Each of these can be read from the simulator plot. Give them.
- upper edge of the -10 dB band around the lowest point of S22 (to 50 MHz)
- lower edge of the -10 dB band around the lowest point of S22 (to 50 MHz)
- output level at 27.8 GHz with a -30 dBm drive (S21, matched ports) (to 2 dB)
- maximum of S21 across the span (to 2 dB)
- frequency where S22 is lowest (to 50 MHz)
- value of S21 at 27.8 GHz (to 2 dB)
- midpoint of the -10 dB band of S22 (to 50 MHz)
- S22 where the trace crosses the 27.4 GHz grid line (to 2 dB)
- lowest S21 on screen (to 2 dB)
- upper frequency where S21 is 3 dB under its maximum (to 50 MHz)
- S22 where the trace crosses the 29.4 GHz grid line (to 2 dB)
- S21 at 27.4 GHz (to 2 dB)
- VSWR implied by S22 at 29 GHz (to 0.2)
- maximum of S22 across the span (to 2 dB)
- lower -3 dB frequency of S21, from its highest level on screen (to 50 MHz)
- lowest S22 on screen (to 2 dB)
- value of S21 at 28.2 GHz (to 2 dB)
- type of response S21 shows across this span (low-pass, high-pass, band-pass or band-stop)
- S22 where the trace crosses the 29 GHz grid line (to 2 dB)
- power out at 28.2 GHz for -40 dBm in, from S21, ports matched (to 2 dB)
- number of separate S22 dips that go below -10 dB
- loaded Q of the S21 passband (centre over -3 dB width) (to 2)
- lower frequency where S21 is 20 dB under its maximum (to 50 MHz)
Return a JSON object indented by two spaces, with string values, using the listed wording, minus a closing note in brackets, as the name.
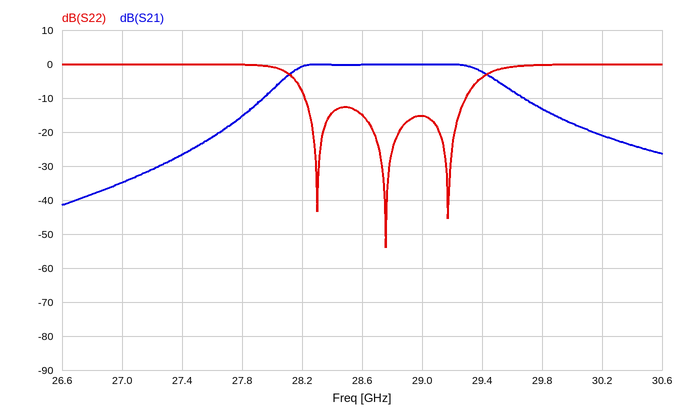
{
  "upper edge of the -10 dB band around the lowest point of S22": "29.30 GHz",
  "lower edge of the -10 dB band around the lowest point of S22": "28.20 GHz",
  "output level at 27.8 GHz with a -30 dBm drive (S21, matched ports)": "-46 dBm",
  "maximum of S21 across the span": "0 dB",
  "frequency where S22 is lowest": "28.75 GHz",
  "value of S21 at 27.8 GHz": "-16 dB",
  "midpoint of the -10 dB band of S22": "28.75 GHz",
  "S22 where the trace crosses the 27.4 GHz grid line": "0 dB",
  "lowest S21 on screen": "-42 dB",
  "upper frequency where S21 is 3 dB under its maximum": "29.45 GHz",
  "S22 where the trace crosses the 29.4 GHz grid line": "-4 dB",
  "S21 at 27.4 GHz": "-26 dB",
  "VSWR implied by S22 at 29 GHz": "1.4",
  "maximum of S22 across the span": "0 dB",
  "lower -3 dB frequency of S21, from its highest level on screen": "28.10 GHz",
  "lowest S22 on screen": "-54 dB",
  "value of S21 at 28.2 GHz": "0 dB",
  "type of response S21 shows across this span": "band-pass",
  "S22 where the trace crosses the 29 GHz grid line": "-16 dB",
  "power out at 28.2 GHz for -40 dBm in, from S21, ports matched": "-40 dBm",
  "number of separate S22 dips that go below -10 dB": "3",
  "loaded Q of the S21 passband (centre over -3 dB width)": "22",
  "lower frequency where S21 is 20 dB under its maximum": "27.65 GHz"
}
